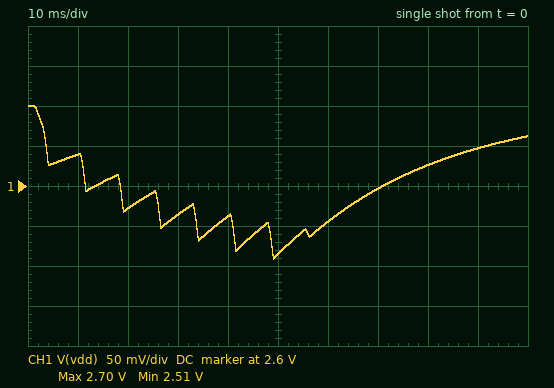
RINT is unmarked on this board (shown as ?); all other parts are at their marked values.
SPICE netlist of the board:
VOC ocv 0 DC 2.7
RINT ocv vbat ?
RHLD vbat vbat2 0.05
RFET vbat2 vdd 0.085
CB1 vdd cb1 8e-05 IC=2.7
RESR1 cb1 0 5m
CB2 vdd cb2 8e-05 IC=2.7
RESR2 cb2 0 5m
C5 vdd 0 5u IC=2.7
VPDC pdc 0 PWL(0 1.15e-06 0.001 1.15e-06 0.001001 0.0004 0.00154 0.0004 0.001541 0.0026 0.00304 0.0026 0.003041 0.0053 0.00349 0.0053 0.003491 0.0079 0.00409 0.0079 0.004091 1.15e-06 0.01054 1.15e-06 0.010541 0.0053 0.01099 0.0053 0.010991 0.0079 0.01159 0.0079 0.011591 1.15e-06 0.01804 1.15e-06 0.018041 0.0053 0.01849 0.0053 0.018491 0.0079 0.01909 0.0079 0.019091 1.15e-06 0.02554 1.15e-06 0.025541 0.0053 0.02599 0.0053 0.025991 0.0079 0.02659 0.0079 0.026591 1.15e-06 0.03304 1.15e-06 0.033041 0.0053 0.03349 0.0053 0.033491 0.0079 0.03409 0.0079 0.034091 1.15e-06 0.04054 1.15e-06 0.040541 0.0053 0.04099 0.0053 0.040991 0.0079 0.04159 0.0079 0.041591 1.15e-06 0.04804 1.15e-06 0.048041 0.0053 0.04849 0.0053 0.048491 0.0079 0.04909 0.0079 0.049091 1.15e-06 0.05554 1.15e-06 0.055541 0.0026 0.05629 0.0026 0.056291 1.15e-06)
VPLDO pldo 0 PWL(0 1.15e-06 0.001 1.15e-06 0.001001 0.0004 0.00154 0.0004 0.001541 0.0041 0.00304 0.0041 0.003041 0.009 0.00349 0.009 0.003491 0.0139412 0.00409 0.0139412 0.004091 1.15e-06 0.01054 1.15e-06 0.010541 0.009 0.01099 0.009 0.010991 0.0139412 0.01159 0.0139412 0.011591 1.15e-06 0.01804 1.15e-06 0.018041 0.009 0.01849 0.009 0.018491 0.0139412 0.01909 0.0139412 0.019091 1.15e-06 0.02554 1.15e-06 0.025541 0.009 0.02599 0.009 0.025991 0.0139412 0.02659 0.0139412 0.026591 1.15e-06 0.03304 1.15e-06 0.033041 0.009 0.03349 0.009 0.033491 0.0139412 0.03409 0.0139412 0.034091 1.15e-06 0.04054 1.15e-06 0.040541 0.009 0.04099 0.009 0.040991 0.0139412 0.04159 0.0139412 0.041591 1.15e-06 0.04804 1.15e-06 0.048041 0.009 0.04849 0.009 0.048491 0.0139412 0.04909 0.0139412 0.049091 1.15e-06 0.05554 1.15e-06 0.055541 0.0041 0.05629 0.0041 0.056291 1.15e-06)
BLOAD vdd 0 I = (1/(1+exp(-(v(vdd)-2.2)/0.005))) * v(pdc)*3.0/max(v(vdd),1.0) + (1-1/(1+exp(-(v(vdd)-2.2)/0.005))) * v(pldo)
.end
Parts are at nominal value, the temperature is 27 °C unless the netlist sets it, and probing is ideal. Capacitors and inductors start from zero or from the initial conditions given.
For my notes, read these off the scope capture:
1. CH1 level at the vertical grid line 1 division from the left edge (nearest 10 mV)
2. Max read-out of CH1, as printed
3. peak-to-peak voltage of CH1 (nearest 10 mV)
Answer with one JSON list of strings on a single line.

["2.64 V", "2.70 V", "190 mV"]
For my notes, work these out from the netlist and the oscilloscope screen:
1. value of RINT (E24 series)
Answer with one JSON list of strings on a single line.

["180 Ω"]
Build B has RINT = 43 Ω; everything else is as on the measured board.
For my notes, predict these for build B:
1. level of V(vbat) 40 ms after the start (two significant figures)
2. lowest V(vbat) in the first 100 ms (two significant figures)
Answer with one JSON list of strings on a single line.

["2.7 V", "2.6 V"]
